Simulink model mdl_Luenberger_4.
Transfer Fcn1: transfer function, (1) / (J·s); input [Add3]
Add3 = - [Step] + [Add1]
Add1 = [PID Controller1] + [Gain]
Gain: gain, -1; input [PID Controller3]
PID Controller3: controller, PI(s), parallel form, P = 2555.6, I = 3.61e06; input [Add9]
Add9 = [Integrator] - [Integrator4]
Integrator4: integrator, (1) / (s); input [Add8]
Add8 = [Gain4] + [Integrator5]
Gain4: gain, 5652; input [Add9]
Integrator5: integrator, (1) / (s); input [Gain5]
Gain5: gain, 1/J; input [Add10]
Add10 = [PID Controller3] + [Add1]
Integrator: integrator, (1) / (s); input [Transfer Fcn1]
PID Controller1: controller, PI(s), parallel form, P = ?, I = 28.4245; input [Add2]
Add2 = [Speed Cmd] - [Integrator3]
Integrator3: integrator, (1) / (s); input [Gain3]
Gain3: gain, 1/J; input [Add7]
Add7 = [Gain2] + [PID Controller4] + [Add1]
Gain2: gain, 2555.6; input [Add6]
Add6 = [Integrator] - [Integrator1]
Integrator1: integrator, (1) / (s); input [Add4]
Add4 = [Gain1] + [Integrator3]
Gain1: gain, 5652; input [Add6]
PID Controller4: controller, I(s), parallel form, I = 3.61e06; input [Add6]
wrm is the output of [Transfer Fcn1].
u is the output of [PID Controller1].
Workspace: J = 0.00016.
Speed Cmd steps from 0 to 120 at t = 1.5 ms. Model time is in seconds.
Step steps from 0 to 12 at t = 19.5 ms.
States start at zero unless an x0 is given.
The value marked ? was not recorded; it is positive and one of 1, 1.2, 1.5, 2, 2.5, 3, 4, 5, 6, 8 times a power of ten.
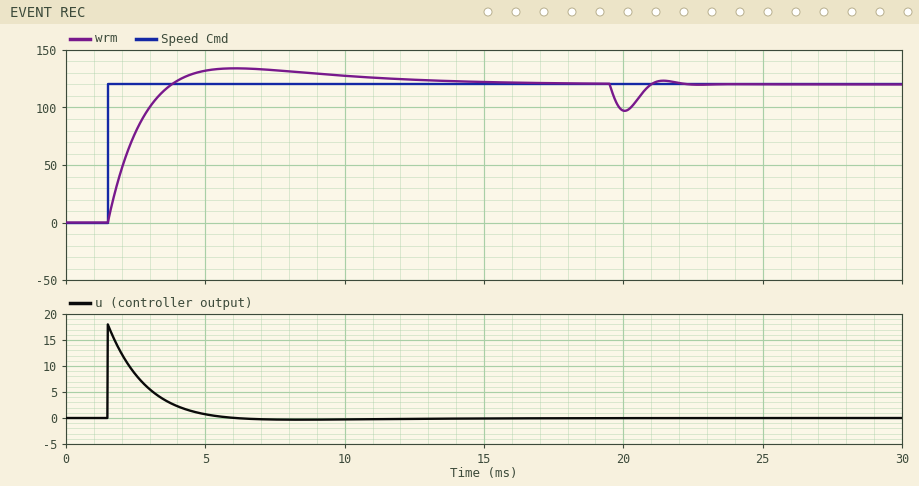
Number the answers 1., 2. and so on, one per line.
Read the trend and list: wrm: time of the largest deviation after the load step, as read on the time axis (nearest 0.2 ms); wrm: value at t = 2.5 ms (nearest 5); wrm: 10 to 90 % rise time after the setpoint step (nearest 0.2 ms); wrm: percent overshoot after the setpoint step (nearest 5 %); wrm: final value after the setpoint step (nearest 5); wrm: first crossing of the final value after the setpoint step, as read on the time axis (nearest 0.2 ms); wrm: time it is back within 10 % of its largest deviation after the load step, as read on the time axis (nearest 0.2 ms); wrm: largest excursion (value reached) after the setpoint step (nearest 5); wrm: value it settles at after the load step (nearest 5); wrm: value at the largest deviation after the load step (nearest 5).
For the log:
1. 20.0 ms
2. 80
3. 1.6 ms
4. 10 %
5. 120
6. 3.8 ms
7. 21.8 ms
8. 135
9. 120
10. 95
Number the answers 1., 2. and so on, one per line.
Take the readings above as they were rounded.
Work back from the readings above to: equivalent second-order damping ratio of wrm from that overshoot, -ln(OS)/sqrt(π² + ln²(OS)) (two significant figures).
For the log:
1. 0.59
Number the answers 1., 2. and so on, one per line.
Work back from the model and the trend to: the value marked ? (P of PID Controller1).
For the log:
1. 0.15
